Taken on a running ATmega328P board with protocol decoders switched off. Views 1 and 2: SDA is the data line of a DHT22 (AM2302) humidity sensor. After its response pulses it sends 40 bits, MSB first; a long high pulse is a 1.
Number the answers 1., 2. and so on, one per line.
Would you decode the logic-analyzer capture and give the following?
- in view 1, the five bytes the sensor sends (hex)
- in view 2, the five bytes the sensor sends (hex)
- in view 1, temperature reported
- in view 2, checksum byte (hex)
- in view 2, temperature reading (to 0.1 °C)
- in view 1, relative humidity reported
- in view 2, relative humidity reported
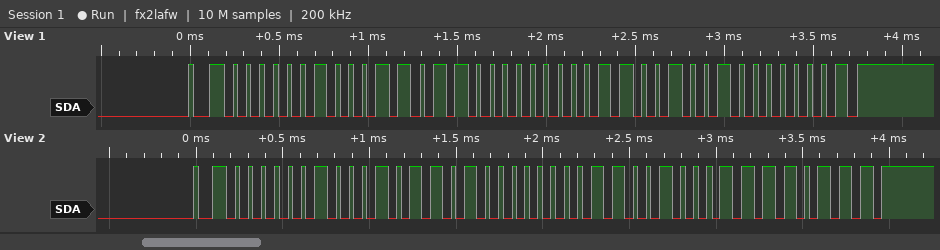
1. 02 36 00 C9 01
2. 02 2D 00 C8 F7
3. 20.1 °C
4. 0xF7
5. 20.0 °C
6. 56.6 %
7. 55.7 %
